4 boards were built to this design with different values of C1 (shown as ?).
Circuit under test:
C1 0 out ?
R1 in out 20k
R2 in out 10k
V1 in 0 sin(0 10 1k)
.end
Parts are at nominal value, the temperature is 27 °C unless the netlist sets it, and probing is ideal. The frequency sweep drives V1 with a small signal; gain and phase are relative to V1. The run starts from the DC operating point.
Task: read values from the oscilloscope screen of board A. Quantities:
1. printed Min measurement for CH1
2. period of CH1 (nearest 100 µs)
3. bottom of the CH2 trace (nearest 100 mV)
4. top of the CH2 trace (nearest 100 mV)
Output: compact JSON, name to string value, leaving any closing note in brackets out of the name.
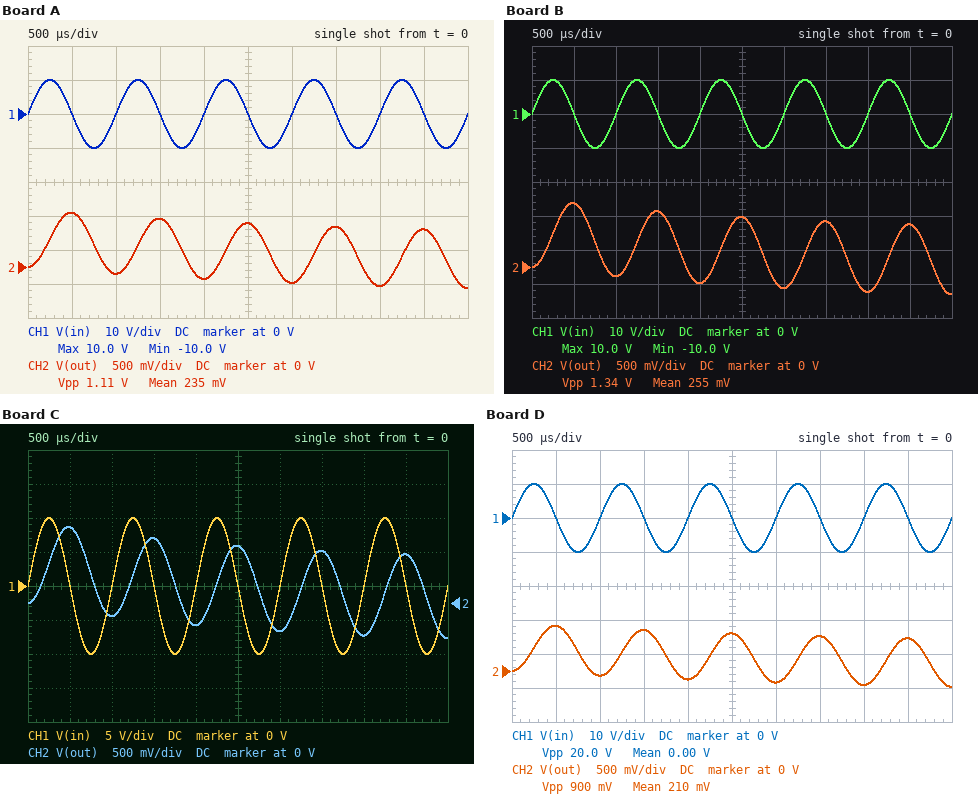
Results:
{"printed Min measurement for CH1": "-10.0 V", "period of CH1": "1.0 ms", "bottom of the CH2 trace": "-300 mV", "top of the CH2 trace": "800 mV"}
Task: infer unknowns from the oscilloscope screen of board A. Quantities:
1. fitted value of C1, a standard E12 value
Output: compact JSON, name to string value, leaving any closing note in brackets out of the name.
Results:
{"fitted value of C1, a standard E12 value": "560 nF"}
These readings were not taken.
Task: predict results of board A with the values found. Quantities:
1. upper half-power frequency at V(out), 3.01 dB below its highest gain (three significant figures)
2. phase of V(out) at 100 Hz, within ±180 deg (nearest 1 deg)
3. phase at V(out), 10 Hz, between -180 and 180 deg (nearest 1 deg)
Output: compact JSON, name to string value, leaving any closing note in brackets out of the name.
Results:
{"upper half-power frequency at V(out), 3.01 dB below its highest gain": "42.6 Hz", "phase of V(out) at 100 Hz, within ±180 deg": "-67 deg", "phase at V(out), 10 Hz, between -180 and 180 deg": "-13 deg"}
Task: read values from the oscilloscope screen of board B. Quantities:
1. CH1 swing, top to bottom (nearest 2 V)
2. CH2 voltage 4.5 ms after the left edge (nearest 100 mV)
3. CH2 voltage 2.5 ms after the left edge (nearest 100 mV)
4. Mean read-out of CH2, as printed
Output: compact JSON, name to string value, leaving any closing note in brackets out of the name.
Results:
{"CH1 swing, top to bottom": "20 V", "CH2 voltage 4.5 ms after the left edge": "600 mV", "CH2 voltage 2.5 ms after the left edge": "700 mV", "Mean read-out of CH2, as printed": "255 mV"}
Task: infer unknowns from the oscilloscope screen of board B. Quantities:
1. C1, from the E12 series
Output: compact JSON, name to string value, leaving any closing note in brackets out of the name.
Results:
{"C1, from the E12 series": "470 nF"}
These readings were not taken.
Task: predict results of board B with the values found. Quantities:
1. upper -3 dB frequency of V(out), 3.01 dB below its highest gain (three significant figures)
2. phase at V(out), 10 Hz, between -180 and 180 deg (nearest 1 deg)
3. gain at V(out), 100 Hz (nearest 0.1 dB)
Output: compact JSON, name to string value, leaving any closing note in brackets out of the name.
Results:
{"upper -3 dB frequency of V(out), 3.01 dB below its highest gain": "50.8 Hz", "phase at V(out), 10 Hz, between -180 and 180 deg": "-11 deg", "gain at V(out), 100 Hz": "-6.9 dB"}
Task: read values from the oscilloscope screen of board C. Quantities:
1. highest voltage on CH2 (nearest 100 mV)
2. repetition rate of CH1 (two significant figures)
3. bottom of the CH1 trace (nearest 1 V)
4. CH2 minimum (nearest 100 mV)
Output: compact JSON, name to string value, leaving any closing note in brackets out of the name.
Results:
{"highest voltage on CH2": "1.1 V", "repetition rate of CH1": "1.0 kHz", "bottom of the CH1 trace": "-10 V", "CH2 minimum": "-500 mV"}
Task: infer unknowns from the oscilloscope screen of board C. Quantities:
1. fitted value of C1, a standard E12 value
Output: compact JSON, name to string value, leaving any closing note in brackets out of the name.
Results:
{"fitted value of C1, a standard E12 value": "390 nF"}
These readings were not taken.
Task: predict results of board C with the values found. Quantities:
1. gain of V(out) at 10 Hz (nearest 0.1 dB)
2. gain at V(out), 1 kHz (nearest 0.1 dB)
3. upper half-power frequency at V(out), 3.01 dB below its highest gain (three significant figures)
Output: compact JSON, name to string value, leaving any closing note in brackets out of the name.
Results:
{"gain of V(out) at 10 Hz": "-0.1 dB", "gain at V(out), 1 kHz": "-24.3 dB", "upper half-power frequency at V(out), 3.01 dB below its highest gain": "61.2 Hz"}
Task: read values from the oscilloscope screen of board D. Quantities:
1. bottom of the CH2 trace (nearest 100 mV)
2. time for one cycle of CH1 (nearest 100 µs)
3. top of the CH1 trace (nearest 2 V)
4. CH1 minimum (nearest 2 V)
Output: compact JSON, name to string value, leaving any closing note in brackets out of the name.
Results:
{"bottom of the CH2 trace": "-200 mV", "time for one cycle of CH1": "1.0 ms", "top of the CH1 trace": "10 V", "CH1 minimum": "-10 V"}
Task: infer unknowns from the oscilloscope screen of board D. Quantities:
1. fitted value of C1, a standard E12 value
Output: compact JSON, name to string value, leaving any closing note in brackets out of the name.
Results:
{"fitted value of C1, a standard E12 value": "680 nF"}
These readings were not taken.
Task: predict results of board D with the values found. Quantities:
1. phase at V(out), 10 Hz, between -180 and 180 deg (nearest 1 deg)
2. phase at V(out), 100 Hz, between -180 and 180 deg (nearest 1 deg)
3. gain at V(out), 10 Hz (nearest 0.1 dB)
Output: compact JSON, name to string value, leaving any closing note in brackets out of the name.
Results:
{"phase at V(out), 10 Hz, between -180 and 180 deg": "-16 deg", "phase at V(out), 100 Hz, between -180 and 180 deg": "-71 deg", "gain at V(out), 10 Hz": "-0.3 dB"}
